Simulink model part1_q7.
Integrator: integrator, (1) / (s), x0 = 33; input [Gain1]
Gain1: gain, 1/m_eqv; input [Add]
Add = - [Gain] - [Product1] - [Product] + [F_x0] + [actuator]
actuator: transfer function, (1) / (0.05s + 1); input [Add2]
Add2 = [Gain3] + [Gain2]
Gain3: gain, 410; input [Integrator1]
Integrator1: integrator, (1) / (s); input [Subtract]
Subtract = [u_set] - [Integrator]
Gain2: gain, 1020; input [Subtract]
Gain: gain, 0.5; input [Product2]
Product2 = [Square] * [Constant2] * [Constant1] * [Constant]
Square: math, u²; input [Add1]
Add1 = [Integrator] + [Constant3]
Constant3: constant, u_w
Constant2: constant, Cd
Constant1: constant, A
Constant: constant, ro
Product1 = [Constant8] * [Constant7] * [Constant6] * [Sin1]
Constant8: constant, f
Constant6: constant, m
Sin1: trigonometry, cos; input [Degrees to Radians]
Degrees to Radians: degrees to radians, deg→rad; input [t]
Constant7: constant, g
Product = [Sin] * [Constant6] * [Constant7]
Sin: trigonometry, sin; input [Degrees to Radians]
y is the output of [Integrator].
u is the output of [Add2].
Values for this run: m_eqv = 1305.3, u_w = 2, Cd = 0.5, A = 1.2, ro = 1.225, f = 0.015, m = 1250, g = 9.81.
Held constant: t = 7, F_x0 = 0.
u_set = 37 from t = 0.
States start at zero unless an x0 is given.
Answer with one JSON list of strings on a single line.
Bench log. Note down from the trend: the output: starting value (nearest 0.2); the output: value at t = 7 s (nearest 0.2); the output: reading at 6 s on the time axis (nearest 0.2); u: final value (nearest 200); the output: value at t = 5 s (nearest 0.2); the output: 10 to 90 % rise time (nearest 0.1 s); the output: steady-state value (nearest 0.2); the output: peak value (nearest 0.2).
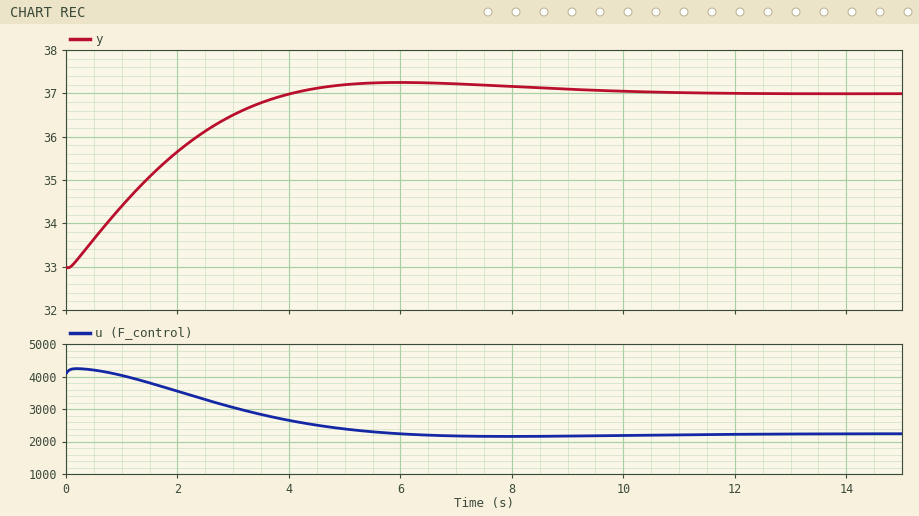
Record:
["33.0", "37.2", "37.2", "2200", "37.2", "2.8 s", "37.0", "37.2"]
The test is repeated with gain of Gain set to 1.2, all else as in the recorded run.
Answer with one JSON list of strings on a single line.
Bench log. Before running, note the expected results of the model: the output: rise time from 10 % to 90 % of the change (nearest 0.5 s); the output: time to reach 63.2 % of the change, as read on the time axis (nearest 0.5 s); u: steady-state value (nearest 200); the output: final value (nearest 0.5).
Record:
["3.5 s", "2.5 s", "3000", "37.0"]
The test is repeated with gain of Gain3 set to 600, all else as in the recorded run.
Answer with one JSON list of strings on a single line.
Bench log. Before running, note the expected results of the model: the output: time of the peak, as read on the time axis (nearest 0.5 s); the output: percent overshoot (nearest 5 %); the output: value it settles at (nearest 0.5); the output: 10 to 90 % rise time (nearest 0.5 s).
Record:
["4.5 s", "15 %", "37.0", "2.0 s"]
